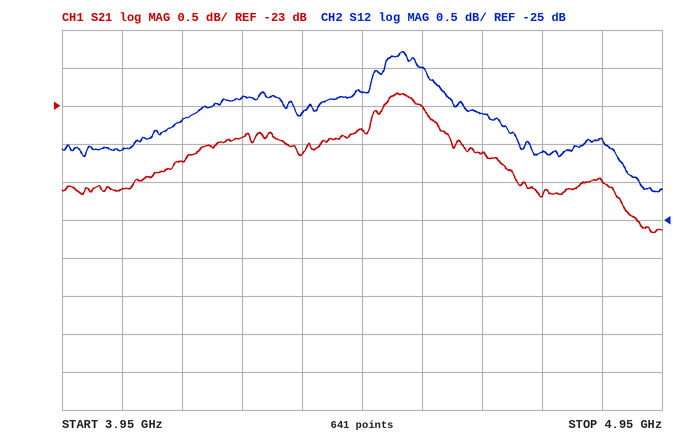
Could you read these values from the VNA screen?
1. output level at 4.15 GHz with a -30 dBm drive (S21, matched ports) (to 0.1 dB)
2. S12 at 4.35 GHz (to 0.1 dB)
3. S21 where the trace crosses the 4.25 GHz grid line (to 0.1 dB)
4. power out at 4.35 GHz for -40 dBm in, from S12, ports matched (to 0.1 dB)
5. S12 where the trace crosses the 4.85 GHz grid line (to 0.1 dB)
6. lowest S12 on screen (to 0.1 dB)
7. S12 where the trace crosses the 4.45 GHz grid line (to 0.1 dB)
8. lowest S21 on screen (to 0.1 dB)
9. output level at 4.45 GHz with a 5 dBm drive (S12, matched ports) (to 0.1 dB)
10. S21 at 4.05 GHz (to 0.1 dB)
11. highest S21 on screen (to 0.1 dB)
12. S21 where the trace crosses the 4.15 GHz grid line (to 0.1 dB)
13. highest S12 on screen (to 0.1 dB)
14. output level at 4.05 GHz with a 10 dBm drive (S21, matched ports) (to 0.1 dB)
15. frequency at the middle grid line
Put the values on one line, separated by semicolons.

-53.7 dBm; -23.6 dB; -23.4 dB; -63.6 dBm; -23.9 dB; -24.6 dB; -23.3 dB; -24.7 dB; -18.3 dBm; -24.1 dB; -22.8 dB; -23.7 dB; -22.8 dB; -14.1 dBm; 4.45 GHz
